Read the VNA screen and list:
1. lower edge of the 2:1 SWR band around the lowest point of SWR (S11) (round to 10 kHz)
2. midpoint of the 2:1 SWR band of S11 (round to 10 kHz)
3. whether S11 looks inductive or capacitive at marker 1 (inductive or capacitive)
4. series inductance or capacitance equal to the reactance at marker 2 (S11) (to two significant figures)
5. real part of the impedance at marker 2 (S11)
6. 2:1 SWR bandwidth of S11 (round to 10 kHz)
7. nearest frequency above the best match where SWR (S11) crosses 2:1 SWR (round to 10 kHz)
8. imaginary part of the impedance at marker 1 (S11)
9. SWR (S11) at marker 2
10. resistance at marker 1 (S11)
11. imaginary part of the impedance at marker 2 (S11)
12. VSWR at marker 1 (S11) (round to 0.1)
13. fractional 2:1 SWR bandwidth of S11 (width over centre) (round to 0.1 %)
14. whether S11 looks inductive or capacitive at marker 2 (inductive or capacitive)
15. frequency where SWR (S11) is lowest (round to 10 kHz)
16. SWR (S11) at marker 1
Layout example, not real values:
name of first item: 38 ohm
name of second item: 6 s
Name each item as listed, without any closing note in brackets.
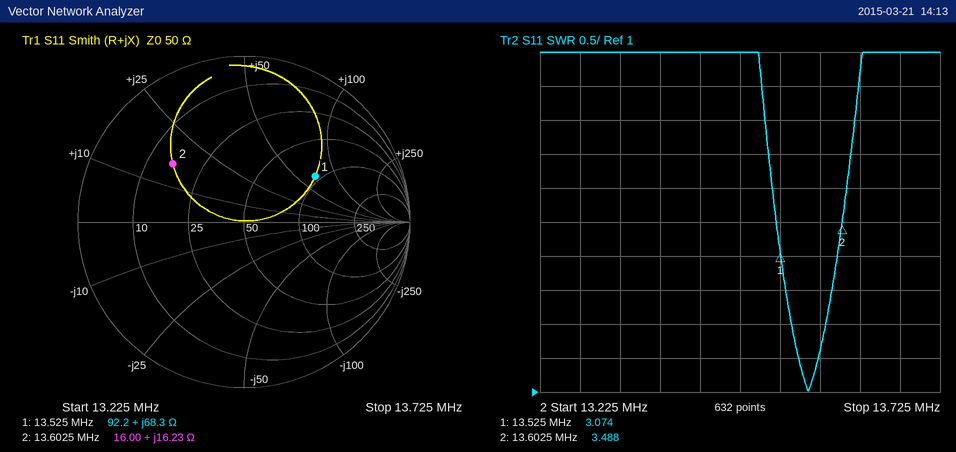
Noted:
lower edge of the 2:1 SWR band around the lowest point of SWR (S11): 13.54 MHz
midpoint of the 2:1 SWR band of S11: 13.56 MHz
whether S11 looks inductive or capacitive at marker 1: inductive
series inductance or capacitance equal to the reactance at marker 2 (S11): 190 nH
real part of the impedance at marker 2: 16.00 Ω
2:1 SWR bandwidth of S11: 40 kHz
nearest frequency above the best match where SWR (S11) crosses 2:1 SWR: 13.58 MHz
imaginary part of the impedance at marker 1: +68.3 Ω
SWR (S11) at marker 2: 3.488
resistance at marker 1: 92.2 Ω
imaginary part of the impedance at marker 2: +16.23 Ω
VSWR at marker 1 (S11): 3.1
fractional 2:1 SWR bandwidth of S11 (width over centre): 0.3 %
whether S11 looks inductive or capacitive at marker 2: inductive
frequency where SWR (S11) is lowest: 13.56 MHz
SWR (S11) at marker 1: 3.074
